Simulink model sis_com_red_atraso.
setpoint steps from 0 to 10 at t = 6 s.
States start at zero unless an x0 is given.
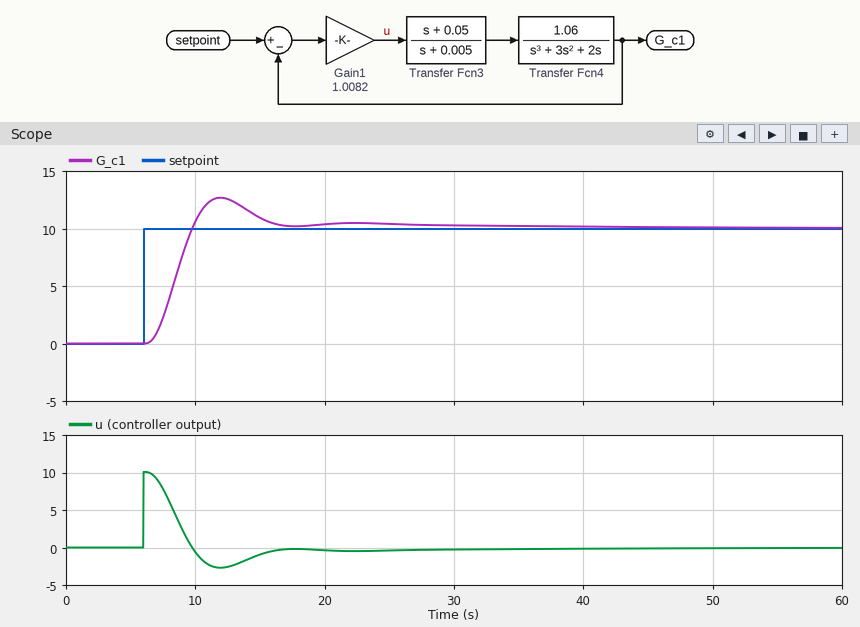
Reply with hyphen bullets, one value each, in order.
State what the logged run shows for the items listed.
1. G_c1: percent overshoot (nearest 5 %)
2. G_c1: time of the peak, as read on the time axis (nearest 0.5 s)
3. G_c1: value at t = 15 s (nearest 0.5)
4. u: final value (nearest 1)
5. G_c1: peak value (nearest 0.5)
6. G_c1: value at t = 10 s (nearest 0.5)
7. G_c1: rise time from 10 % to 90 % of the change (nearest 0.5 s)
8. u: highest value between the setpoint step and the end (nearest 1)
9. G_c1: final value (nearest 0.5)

- 25 %
- 12.0 s
- 11.0
- 0
- 12.5
- 10.5
- 2.5 s
- 10
- 10.0
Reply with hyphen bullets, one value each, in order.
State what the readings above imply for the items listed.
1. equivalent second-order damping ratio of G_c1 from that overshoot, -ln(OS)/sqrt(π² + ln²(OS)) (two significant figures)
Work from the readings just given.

- 0.40
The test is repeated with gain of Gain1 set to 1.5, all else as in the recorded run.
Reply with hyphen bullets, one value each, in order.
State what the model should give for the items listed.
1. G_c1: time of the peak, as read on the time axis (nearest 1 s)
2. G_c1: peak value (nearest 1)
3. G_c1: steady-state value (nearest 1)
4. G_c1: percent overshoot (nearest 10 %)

- 11 s
- 14
- 10
- 40 %
